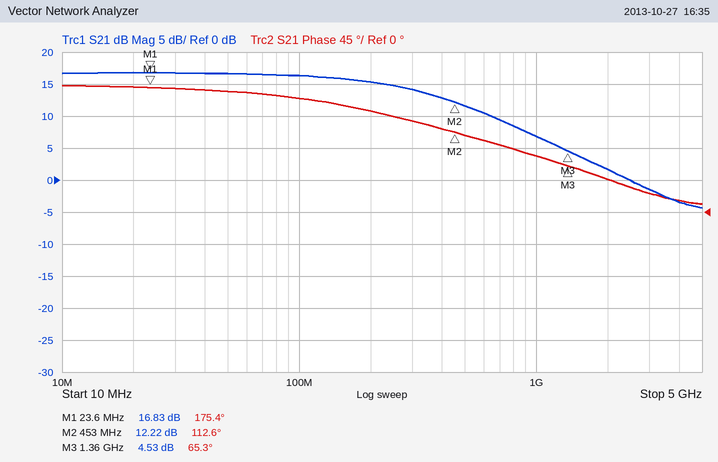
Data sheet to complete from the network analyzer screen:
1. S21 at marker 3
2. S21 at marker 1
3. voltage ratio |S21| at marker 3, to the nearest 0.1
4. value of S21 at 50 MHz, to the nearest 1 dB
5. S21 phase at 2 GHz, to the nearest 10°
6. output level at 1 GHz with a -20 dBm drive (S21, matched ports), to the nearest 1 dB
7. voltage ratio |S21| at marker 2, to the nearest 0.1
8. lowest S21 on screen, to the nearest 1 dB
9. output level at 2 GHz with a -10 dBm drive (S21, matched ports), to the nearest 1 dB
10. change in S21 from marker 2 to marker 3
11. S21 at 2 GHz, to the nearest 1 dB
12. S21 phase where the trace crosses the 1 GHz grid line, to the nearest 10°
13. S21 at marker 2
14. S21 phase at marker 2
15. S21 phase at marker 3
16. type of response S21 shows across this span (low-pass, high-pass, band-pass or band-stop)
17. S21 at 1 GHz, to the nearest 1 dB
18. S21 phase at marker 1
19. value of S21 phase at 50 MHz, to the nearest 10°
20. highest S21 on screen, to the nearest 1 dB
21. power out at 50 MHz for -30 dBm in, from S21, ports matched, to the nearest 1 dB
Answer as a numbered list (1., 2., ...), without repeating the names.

1. 4.53 dB
2. 16.83 dB
3. 1.7
4. 17 dB
5. 50°
6. -13 dBm
7. 4.1
8. -4 dB
9. -8 dBm
10. -7.69 dB
11. 2 dB
12. 80°
13. 12.22 dB
14. 112.6°
15. 65.3°
16. low-pass
17. 7 dB
18. 175.4°
19. 170°
20. 17 dB
21. -13 dBm
